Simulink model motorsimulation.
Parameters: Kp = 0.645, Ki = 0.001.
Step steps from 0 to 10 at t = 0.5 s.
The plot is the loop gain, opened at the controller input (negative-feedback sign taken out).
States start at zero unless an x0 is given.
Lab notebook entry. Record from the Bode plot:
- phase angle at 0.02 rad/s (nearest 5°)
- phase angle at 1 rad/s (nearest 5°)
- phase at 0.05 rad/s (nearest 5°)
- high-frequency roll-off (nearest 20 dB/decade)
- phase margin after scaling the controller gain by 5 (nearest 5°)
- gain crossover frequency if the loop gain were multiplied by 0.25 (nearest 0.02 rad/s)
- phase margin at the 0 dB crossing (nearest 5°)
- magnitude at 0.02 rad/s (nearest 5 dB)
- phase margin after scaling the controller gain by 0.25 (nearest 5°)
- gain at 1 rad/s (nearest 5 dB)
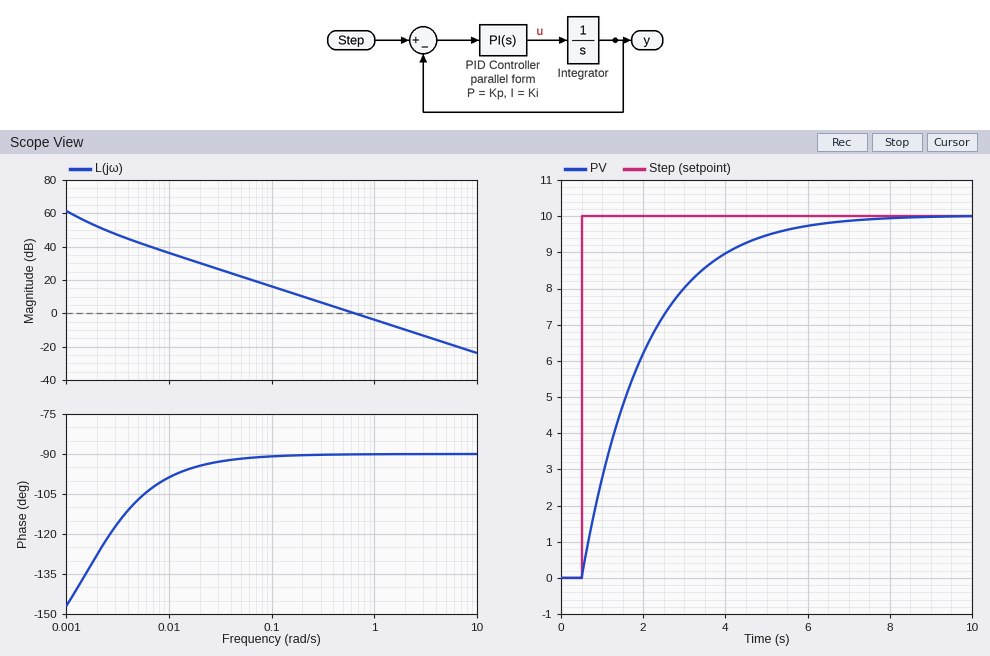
-95°
-90°
-90°
-20 dB/decade
90°
0.16 rad/s
90°
30 dB
90°
-5 dB
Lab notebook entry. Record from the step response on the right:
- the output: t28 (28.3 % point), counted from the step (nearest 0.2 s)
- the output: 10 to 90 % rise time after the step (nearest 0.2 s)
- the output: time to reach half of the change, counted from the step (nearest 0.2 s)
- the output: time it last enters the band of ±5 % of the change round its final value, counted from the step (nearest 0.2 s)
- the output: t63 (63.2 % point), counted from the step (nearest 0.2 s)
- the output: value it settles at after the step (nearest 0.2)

0.6 s
3.4 s
1.0 s
4.6 s
1.6 s
10.0
